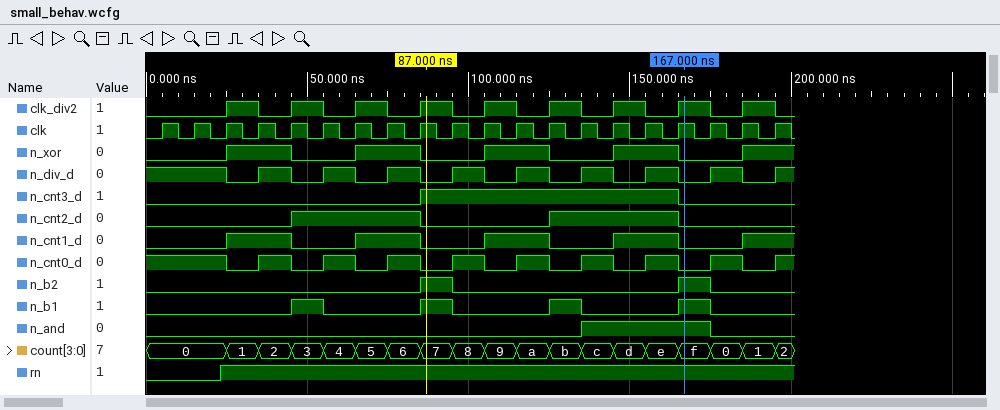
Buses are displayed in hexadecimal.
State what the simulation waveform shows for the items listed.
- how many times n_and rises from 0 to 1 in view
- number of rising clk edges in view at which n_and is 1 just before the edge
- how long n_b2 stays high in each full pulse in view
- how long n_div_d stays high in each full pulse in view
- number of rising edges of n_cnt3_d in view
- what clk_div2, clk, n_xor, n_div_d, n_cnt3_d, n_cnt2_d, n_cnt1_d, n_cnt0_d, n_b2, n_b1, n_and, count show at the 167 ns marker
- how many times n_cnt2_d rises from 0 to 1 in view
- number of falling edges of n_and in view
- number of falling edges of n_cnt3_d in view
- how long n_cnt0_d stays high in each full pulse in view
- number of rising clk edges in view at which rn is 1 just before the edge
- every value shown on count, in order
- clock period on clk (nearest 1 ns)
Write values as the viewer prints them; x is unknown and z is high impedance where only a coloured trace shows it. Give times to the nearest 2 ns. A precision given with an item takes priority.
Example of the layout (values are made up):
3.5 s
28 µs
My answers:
1
4
10 ns, 10 ns
10 ns, 10 ns, 10 ns, 10 ns, 10 ns, 10 ns, 10 ns, 10 ns
1
clk_div2=1, clk=1, n_xor=0, n_div_d=0, n_cnt3_d=0, n_cnt2_d=0, n_cnt1_d=0, n_cnt0_d=0, n_b2=1, n_b1=1, n_and=1, count=f
2
1
1
10 ns, 10 ns, 10 ns, 10 ns, 10 ns, 10 ns, 10 ns, 10 ns
18
0, 1, 2, 3, 4, 5, 6, 7, 8, 9, a, b, c, d, e, f, 0, 1, 2
10 ns
